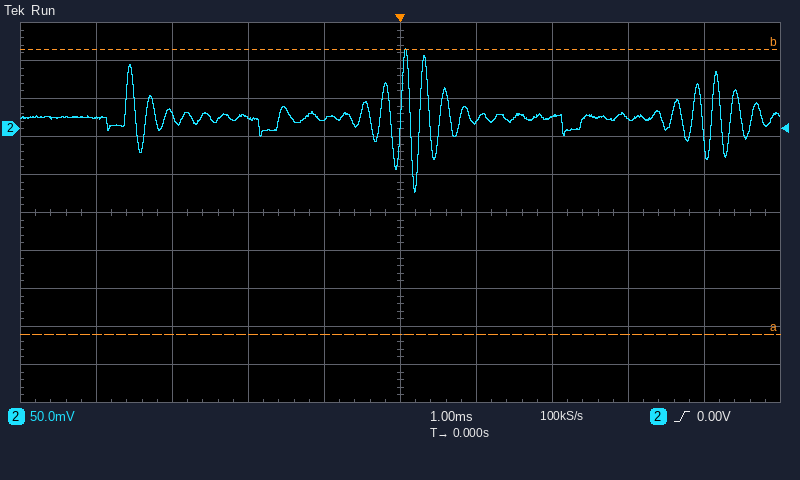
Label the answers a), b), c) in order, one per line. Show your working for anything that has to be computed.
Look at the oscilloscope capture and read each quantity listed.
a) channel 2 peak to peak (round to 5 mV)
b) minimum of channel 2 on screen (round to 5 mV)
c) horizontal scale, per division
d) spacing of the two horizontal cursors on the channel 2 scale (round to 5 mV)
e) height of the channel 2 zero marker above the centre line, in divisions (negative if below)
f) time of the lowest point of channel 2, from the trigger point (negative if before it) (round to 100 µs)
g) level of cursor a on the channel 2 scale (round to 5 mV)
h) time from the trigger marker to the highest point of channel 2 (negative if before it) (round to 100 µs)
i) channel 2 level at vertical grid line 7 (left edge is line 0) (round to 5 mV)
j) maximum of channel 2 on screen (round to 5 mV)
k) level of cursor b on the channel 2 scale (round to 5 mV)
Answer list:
a) 105 mV − (-85 mV) = 190 mV
b) -85 mV
c) 1 ms
d) 375 mV
e) +2.2 div
f) +200 µs
g) -270 mV
h) +100 µs
i) 15 mV
j) 105 mV
k) 105 mV
